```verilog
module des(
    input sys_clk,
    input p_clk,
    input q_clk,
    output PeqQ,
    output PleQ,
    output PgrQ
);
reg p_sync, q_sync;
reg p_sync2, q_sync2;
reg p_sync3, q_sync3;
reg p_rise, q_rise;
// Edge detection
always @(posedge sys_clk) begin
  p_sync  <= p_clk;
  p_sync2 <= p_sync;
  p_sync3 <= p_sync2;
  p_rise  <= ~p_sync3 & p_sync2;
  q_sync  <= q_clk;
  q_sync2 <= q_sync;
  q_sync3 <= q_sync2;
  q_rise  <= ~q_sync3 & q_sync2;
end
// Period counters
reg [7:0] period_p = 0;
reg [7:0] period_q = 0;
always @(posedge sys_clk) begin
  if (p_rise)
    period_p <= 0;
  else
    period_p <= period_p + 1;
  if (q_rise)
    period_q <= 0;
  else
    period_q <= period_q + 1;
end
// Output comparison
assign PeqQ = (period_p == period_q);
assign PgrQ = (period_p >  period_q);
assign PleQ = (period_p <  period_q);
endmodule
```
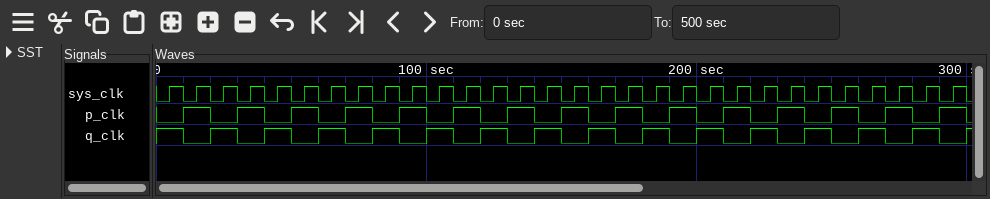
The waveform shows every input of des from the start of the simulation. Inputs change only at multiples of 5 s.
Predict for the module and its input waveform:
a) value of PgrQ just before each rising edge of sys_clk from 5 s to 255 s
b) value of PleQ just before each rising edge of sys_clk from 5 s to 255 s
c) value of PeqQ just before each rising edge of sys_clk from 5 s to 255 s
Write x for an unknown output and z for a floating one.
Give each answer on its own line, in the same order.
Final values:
0 0 0 0 0 0 1 0 1 0 1 0 1 0 1 0 1 0 1 0 1 0 1 0 1 0
0 0 0 0 0 1 0 1 0 1 0 1 0 1 0 1 0 1 0 1 0 1 0 1 0 1
1 1 1 1 1 0 0 0 0 0 0 0 0 0 0 0 0 0 0 0 0 0 0 0 0 0
